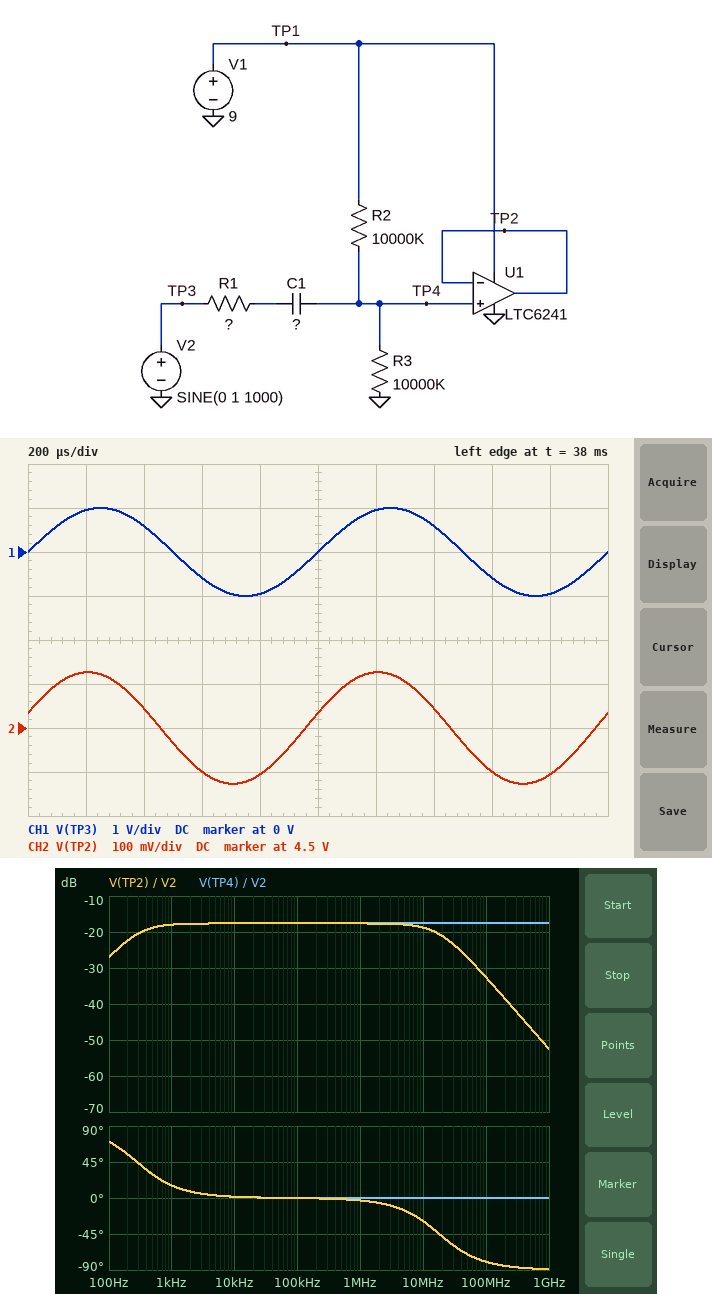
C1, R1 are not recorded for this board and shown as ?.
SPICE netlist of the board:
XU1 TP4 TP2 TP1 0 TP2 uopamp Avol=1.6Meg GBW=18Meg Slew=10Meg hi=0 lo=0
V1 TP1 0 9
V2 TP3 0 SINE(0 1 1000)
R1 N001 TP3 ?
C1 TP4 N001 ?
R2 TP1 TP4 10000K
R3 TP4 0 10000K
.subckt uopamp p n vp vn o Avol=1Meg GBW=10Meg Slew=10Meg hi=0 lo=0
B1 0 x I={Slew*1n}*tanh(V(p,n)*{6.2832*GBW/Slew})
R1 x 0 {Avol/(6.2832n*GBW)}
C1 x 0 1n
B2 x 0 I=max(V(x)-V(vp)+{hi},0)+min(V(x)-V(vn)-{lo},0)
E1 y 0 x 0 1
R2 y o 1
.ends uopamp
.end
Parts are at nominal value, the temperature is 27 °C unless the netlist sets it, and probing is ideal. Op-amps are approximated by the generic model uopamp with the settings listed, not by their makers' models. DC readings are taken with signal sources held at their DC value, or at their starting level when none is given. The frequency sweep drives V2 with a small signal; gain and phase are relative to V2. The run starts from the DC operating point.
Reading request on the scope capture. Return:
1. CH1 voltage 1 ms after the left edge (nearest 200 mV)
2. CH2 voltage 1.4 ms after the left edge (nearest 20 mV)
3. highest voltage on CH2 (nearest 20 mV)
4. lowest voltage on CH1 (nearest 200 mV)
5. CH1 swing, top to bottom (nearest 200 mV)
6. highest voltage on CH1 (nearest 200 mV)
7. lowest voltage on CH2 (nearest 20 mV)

0 V
4.54 V
4.62 V
-1.0 V
2.0 V
1.0 V
4.38 V
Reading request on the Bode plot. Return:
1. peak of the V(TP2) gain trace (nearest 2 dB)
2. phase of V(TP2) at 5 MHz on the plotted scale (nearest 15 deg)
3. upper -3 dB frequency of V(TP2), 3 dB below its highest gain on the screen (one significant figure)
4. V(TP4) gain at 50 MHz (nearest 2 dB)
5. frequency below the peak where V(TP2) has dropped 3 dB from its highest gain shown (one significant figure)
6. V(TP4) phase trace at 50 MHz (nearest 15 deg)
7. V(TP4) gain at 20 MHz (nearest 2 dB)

-18 dB
-15 deg
20 MHz
-18 dB
300 Hz
0 deg
-18 dB
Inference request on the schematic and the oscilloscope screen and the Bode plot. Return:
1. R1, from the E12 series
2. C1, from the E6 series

33 MΩ
15 pF
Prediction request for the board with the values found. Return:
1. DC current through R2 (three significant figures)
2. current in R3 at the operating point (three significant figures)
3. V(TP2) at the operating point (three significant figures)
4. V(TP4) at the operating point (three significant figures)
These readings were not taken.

450 nA
450 nA
4.50 V
4.50 V
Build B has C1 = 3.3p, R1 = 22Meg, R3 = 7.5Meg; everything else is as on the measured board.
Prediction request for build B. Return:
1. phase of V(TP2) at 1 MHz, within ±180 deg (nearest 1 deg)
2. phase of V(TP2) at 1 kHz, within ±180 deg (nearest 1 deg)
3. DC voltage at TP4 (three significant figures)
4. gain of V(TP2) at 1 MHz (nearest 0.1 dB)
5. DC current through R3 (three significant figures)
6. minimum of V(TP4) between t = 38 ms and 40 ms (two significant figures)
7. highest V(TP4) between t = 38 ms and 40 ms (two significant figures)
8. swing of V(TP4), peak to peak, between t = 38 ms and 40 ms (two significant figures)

-3 deg
61 deg
3.86 V
-15.8 dB
514 nA
3.8 V
3.9 V
160 mV
